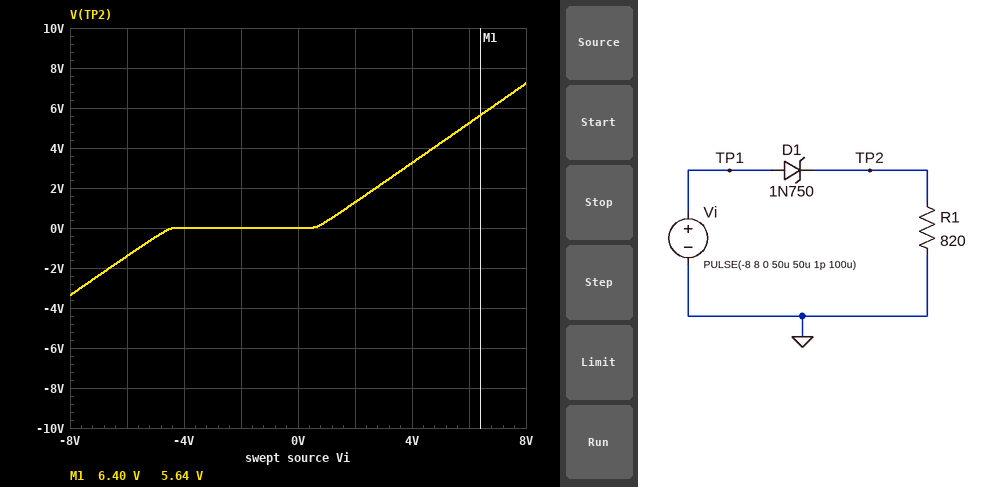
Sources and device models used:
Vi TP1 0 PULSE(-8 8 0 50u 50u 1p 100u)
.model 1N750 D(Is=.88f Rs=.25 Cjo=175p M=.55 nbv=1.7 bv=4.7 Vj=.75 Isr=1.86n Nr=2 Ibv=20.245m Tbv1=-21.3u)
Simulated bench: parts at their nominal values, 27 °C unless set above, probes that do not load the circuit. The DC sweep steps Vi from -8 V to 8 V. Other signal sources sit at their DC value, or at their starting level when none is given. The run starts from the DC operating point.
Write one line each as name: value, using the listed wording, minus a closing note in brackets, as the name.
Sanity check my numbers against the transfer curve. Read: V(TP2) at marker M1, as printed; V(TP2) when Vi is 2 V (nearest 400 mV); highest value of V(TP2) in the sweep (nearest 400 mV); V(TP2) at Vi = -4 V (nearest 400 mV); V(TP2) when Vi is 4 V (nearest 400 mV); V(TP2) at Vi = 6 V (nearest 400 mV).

V(TP2) at marker M1, as printed: 5.64 V
V(TP2) when Vi is 2 V: 1.2 V
highest value of V(TP2) in the sweep: 7.2 V
V(TP2) at Vi = -4 V: 0 V
V(TP2) when Vi is 4 V: 3.2 V
V(TP2) at Vi = 6 V: 5.2 V
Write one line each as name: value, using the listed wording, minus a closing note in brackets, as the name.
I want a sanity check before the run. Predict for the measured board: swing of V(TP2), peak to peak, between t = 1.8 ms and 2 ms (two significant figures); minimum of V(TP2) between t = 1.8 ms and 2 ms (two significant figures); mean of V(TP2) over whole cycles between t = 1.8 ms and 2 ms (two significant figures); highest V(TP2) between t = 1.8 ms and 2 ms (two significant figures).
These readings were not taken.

swing of V(TP2), peak to peak, between t = 1.8 ms and 2 ms: 11 V
minimum of V(TP2) between t = 1.8 ms and 2 ms: -3.4 V
mean of V(TP2) over whole cycles between t = 1.8 ms and 2 ms: 1.3 V
highest V(TP2) between t = 1.8 ms and 2 ms: 7.2 V
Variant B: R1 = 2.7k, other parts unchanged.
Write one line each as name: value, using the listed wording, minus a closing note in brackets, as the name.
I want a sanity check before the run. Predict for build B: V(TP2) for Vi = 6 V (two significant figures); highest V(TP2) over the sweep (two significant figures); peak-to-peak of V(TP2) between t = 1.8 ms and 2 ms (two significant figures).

V(TP2) for Vi = 6 V: 5.3 V
highest V(TP2) over the sweep: 7.3 V
peak-to-peak of V(TP2) between t = 1.8 ms and 2 ms: 11 V
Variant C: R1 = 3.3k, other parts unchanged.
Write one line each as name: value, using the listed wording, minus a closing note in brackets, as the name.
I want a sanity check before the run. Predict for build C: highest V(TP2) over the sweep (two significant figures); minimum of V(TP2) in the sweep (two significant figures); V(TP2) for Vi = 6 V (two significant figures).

highest V(TP2) over the sweep: 7.3 V
minimum of V(TP2) in the sweep: -3.4 V
V(TP2) for Vi = 6 V: 5.3 V
